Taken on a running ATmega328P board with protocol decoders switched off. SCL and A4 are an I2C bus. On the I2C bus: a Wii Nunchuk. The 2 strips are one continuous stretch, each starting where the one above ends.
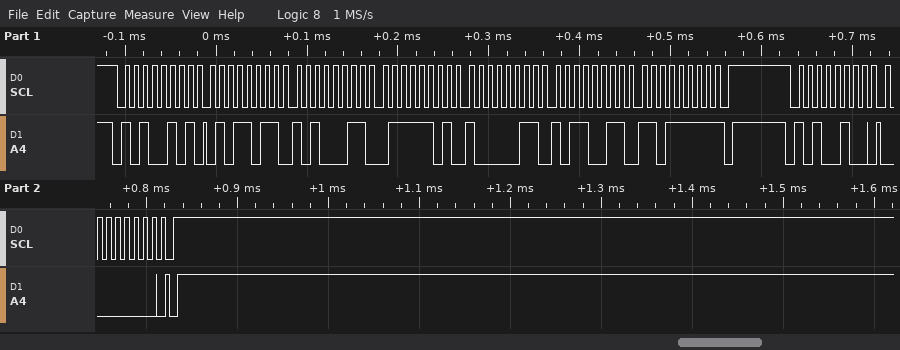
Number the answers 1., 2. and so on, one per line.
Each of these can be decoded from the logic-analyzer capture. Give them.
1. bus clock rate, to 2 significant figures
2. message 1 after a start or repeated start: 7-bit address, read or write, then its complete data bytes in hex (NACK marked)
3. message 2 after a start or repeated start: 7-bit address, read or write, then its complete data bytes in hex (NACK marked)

1. 100 kHz
2. 0x52 read: 5B A3 7D 83 B3 DF NACK
3. 0x52 write: 00
